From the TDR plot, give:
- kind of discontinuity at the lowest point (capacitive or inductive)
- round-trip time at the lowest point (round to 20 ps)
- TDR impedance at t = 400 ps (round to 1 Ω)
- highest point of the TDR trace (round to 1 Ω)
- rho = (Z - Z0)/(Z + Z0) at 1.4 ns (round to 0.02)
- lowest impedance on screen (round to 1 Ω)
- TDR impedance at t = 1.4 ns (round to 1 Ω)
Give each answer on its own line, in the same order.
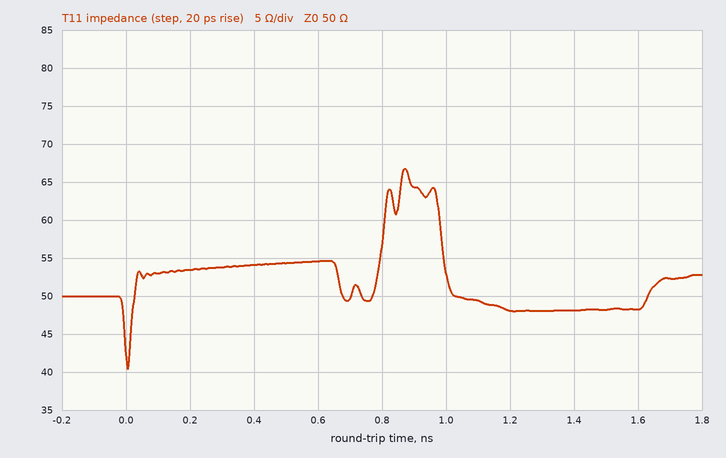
capacitive
0 ps
54 Ω
67 Ω
-0.02
40 Ω
48 Ω
